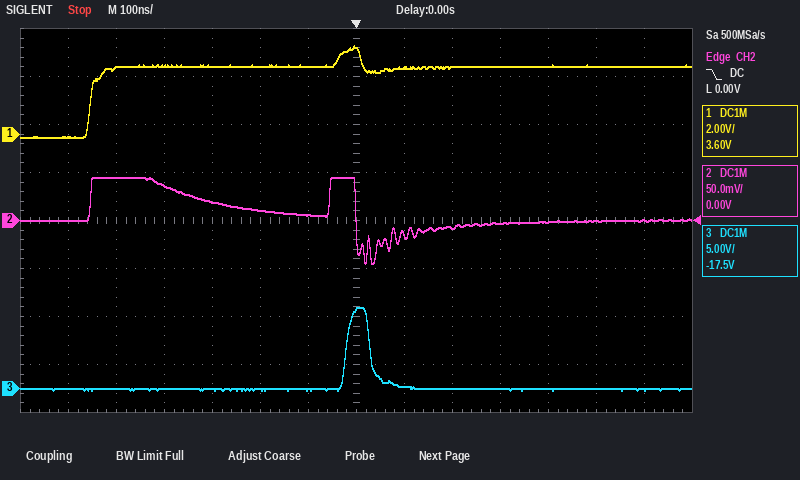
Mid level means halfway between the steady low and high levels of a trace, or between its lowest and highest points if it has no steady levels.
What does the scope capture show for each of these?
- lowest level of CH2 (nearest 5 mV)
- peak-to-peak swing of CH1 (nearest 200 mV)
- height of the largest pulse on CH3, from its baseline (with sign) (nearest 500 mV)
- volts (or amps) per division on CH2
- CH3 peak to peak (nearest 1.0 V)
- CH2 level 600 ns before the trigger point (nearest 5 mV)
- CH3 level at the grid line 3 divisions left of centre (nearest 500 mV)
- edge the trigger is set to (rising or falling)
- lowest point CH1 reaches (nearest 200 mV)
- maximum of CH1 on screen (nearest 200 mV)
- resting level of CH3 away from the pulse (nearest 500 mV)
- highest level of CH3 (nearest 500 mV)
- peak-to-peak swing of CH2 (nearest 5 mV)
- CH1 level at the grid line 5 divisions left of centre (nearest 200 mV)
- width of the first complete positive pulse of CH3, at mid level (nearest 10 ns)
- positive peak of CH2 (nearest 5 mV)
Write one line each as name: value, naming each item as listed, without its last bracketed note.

lowest level of CH2: -45 mV
peak-to-peak swing of CH1: 3.8 V
height of the largest pulse on CH3, from its baseline (with sign): +8.5 V
volts (or amps) per division on CH2: 50 mV
CH3 peak to peak: 9.0 V
CH2 level 600 ns before the trigger point: 0 mV
CH3 level at the grid line 3 divisions left of centre: 0.0 V
edge the trigger is set to: falling
lowest point CH1 reaches: -200 mV
maximum of CH1 on screen: 3.6 V
resting level of CH3 away from the pulse: 0.0 V
highest level of CH3: 8.5 V
peak-to-peak swing of CH2: 90 mV
CH1 level at the grid line 5 divisions left of centre: 2.8 V
width of the first complete positive pulse of CH3, at mid level: 50 ns
positive peak of CH2: 45 mV
